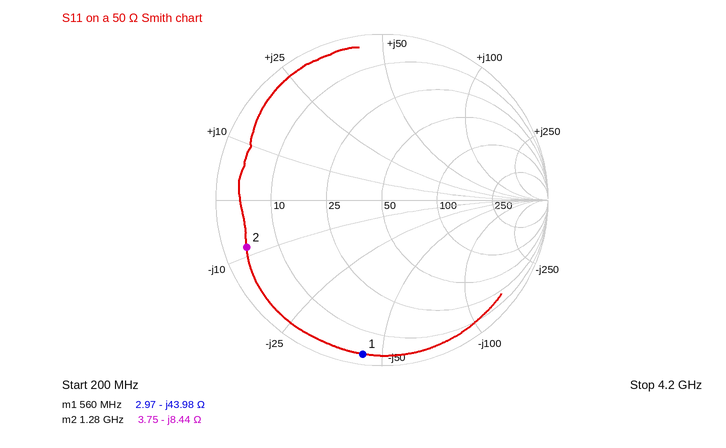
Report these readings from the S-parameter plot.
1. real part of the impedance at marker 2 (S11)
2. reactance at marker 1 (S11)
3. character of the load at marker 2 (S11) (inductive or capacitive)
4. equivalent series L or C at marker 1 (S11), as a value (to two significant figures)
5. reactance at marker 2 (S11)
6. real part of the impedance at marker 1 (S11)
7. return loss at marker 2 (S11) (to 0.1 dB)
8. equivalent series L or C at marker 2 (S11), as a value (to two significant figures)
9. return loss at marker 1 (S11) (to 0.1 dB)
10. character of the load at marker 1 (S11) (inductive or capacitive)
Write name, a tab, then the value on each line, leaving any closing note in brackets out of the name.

real part of the impedance at marker 2	3.75 Ω
reactance at marker 1	-43.98 Ω
character of the load at marker 2 (S11)	capacitive
equivalent series L or C at marker 1 (S11), as a value	6.5 pF
reactance at marker 2	-8.44 Ω
real part of the impedance at marker 1	2.97 Ω
return loss at marker 2 (S11)	1.3 dB
equivalent series L or C at marker 2 (S11), as a value	15 pF
return loss at marker 1 (S11)	0.6 dB
character of the load at marker 1 (S11)	capacitive
